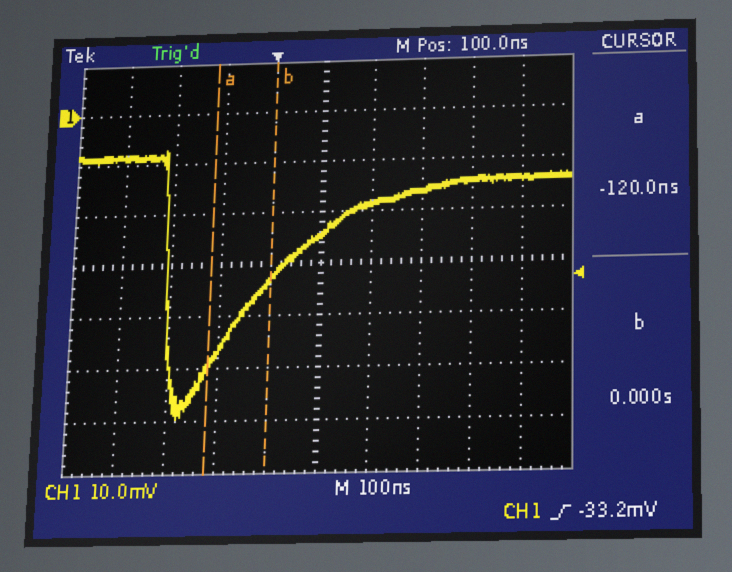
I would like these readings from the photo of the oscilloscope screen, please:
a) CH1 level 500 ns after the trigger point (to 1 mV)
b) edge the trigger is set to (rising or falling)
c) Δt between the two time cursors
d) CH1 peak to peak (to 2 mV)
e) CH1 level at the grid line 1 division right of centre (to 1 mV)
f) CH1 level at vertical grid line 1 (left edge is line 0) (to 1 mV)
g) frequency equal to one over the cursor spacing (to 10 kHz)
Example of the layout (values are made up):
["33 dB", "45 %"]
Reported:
["-14 mV", "rising", "120 ns", "52 mV", "-19 mV", "-9 mV", "8.33 MHz"]
